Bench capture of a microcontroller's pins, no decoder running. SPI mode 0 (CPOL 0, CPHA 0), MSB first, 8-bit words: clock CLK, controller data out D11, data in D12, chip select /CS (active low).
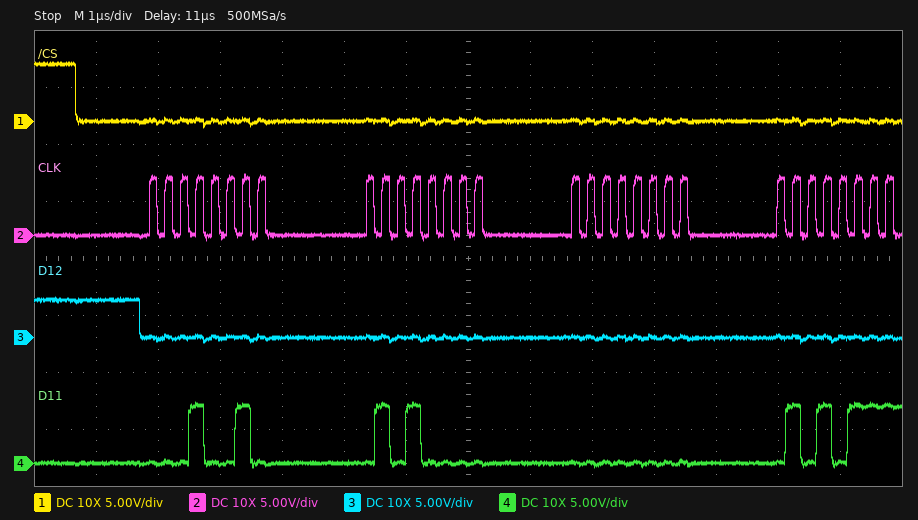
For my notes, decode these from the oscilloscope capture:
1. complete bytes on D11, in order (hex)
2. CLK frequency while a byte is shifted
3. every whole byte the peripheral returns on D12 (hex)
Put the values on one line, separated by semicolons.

12 50 00 57; 4 MHz; 00 00 00 00
